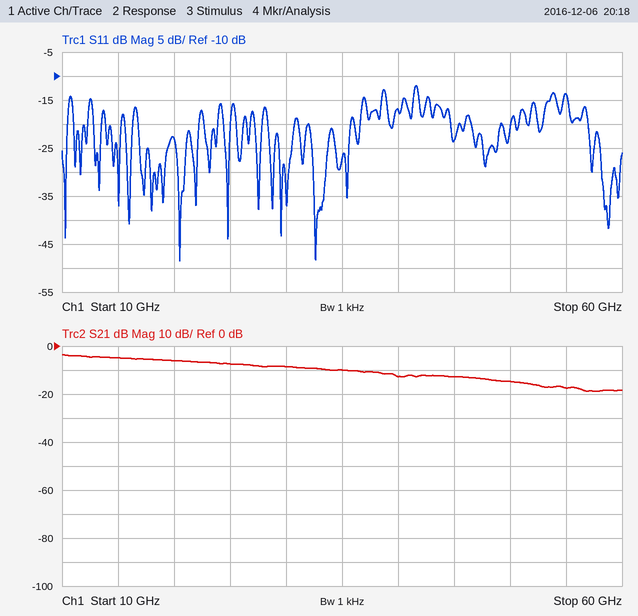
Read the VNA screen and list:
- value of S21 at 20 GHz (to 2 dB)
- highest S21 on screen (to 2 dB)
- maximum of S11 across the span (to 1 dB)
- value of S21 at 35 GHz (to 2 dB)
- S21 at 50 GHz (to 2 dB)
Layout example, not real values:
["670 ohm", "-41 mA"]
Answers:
["-6 dB", "-4 dB", "-12 dB", "-10 dB", "-14 dB"]
